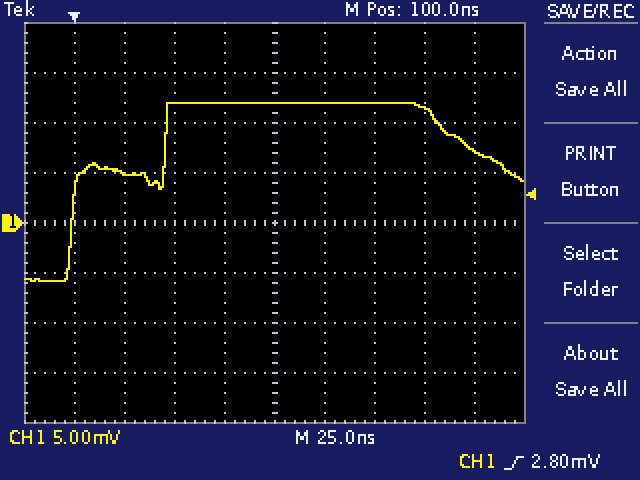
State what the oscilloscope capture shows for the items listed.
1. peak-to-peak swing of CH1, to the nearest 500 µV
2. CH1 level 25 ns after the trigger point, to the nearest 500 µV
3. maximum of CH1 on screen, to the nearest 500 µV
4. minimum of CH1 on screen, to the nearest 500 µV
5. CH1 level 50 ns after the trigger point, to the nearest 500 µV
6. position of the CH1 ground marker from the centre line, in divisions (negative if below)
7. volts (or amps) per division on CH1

18.0 mV
5.0 mV
12.0 mV
-6.0 mV
12.0 mV
0.0 div
5 mV
